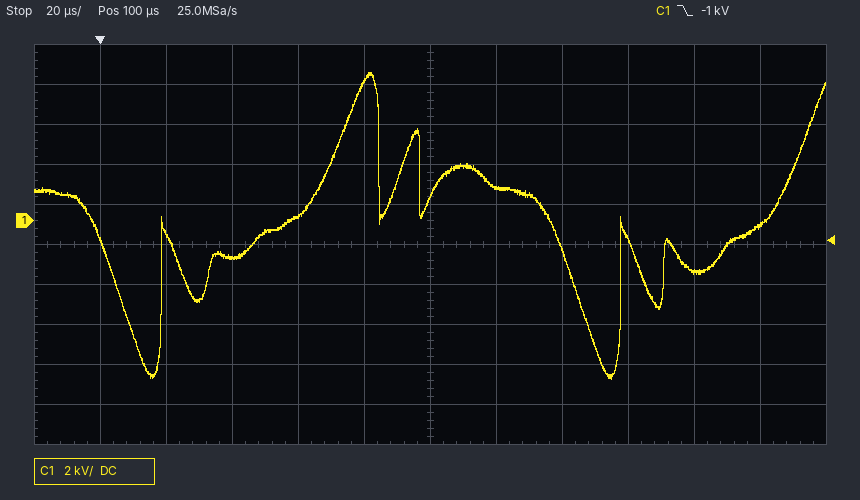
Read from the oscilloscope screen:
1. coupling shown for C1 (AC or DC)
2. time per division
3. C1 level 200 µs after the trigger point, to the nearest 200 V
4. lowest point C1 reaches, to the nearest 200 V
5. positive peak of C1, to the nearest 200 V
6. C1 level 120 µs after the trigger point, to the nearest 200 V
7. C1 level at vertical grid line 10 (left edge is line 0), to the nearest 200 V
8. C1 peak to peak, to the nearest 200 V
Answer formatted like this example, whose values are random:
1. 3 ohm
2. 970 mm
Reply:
1. DC
2. 20 µs
3. -200 V
4. -8.0 kV
5. 7.4 kV
6. 1.6 kV
7. -2.6 kV
8. 15.4 kV
